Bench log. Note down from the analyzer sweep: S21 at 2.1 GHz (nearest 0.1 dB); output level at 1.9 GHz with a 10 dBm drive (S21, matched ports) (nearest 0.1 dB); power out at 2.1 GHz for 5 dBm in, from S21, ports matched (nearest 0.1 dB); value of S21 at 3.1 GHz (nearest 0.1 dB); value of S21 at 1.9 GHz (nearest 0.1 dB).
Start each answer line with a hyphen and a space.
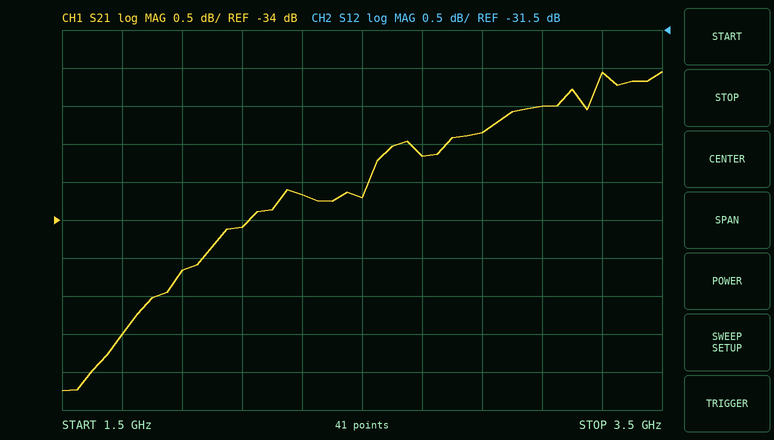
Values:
- -34.1 dB
- -24.7 dBm
- -29.1 dBm
- -32.5 dB
- -34.7 dB
